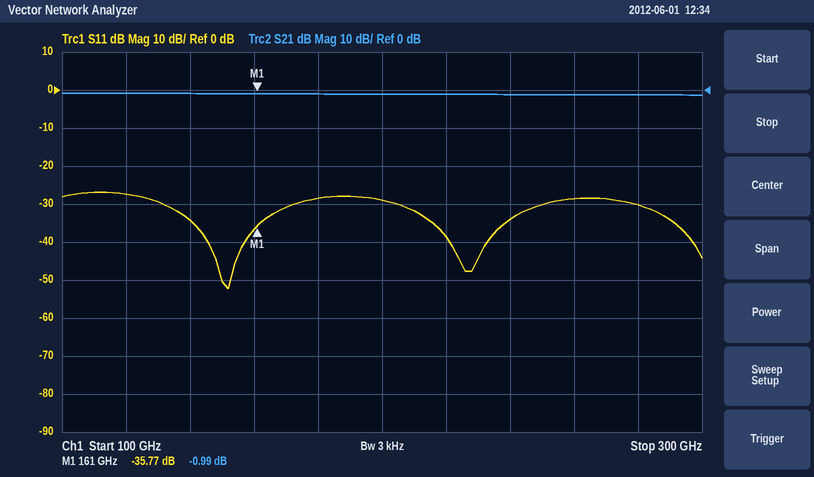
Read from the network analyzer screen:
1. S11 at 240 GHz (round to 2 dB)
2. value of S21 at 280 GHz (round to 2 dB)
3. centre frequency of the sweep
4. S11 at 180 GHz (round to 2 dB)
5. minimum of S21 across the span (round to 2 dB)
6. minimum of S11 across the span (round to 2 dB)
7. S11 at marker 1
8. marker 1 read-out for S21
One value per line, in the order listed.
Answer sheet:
-34 dB
-2 dB
200 GHz
-28 dB
-2 dB
-52 dB
-35.77 dB
-0.99 dB
